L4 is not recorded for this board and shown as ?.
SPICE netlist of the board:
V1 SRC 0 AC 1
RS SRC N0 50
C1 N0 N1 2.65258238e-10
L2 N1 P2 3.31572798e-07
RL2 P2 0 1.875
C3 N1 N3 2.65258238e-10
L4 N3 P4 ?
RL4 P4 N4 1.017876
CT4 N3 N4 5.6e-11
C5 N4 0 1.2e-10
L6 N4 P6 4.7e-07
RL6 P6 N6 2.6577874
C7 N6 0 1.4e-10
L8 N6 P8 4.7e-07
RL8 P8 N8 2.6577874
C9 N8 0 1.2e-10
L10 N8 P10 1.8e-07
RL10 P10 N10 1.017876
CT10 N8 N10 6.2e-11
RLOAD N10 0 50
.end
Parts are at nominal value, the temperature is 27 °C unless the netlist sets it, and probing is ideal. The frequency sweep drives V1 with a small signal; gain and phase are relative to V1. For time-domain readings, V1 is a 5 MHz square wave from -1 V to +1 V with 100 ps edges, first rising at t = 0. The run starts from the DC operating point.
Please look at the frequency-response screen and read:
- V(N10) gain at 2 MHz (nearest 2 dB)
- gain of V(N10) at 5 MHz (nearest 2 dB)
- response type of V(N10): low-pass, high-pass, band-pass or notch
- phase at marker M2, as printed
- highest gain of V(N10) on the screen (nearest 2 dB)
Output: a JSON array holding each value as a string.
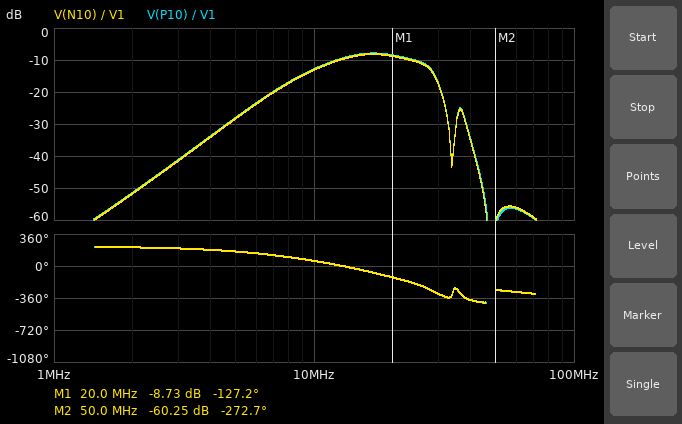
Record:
["-52 dB", "-28 dB", "band-pass", "-272.7 deg", "-8 dB"]
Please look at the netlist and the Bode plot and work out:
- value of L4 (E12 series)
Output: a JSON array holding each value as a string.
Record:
["390 nH"]
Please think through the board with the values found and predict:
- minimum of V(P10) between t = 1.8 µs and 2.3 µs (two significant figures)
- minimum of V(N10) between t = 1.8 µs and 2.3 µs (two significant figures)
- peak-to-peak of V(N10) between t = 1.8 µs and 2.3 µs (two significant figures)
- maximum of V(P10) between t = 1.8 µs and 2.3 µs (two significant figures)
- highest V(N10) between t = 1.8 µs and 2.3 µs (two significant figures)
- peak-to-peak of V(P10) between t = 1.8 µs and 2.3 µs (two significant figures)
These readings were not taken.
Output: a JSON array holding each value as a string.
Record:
["-280 mV", "-270 mV", "540 mV", "280 mV", "270 mV", "550 mV"]
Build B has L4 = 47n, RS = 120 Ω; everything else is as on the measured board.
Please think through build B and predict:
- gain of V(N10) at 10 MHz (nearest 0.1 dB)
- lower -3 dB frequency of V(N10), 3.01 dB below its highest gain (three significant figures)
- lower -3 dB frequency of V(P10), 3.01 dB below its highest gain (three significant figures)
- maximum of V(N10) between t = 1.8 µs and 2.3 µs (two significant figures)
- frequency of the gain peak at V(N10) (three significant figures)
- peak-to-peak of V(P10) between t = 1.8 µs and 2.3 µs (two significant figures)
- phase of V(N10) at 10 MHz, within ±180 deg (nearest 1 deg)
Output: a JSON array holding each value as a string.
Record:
["-19.9 dB", "16.4 MHz", "16.6 MHz", "200 mV", "32.0 MHz", "410 mV", "55 deg"]
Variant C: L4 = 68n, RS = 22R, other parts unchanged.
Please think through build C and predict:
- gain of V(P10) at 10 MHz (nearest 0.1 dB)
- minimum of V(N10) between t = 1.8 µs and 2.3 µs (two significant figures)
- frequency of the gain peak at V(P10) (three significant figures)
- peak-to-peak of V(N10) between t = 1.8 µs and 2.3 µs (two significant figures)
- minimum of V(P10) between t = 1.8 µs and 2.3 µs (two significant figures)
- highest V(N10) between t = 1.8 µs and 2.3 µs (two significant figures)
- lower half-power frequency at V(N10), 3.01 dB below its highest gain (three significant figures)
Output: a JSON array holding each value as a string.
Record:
["-10.7 dB", "-540 mV", "17.1 MHz", "1.1 V", "-560 mV", "540 mV", "12.1 MHz"]
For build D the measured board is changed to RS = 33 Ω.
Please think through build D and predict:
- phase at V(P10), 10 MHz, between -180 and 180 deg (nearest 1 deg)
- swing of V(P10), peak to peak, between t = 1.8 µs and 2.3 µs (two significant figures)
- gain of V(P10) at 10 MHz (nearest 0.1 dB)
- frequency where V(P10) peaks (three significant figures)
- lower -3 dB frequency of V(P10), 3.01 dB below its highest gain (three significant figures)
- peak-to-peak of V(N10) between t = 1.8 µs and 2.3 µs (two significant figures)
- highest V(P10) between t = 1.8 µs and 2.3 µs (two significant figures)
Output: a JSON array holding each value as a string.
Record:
["67 deg", "730 mV", "-11.0 dB", "17.2 MHz", "11.5 MHz", "710 mV", "360 mV"]
